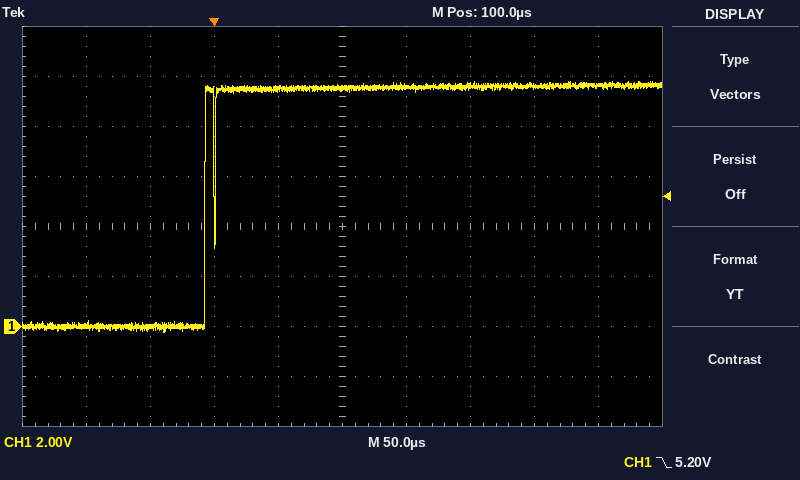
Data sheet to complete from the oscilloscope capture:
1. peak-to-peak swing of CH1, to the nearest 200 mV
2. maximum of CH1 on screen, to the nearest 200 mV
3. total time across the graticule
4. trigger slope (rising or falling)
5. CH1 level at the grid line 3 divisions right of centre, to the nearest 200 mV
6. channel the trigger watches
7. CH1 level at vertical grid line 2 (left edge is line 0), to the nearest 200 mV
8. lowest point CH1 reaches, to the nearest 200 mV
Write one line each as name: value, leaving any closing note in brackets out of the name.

peak-to-peak swing of CH1, to the nearest 200 mV: 10.0 V
maximum of CH1 on screen, to the nearest 200 mV: 9.8 V
total time across the graticule: 500 µs
trigger slope: falling
CH1 level at the grid line 3 divisions right of centre, to the nearest 200 mV: 9.6 V
channel the trigger watches: CH1
CH1 level at vertical grid line 2 (left edge is line 0), to the nearest 200 mV: 0.0 V
lowest point CH1 reaches, to the nearest 200 mV: -200 mV
